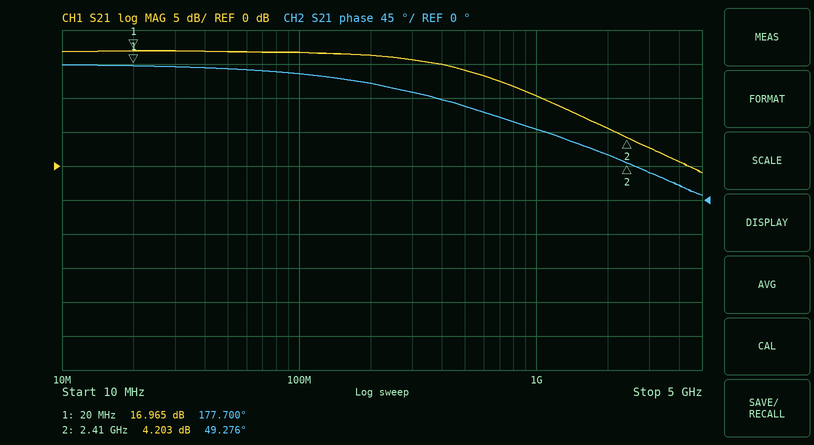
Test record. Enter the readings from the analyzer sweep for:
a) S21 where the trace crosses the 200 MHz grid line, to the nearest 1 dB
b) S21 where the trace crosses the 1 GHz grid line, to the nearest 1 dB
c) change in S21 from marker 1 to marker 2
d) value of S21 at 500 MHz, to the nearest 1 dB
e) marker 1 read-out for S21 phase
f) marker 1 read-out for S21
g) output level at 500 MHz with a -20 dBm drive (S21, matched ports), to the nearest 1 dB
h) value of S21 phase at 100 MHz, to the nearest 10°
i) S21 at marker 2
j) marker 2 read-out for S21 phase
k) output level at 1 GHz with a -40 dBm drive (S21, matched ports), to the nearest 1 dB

16 dB
10 dB
-12.762 dB
14 dB
177.700°
16.965 dB
-6 dBm
170°
4.203 dB
49.276°
-30 dBm
